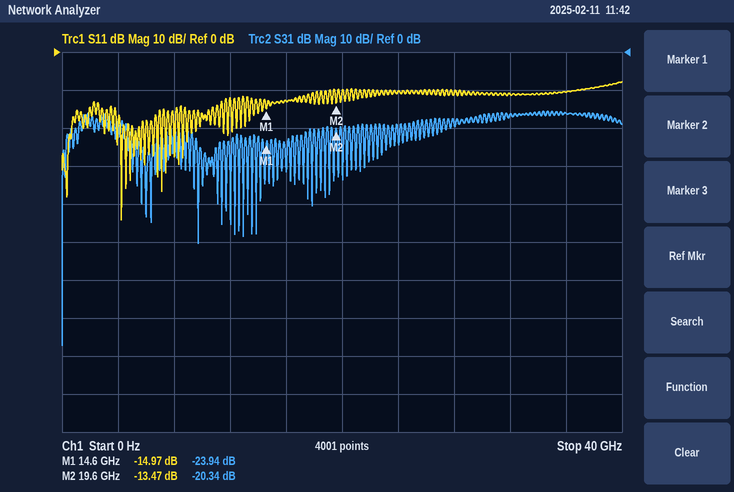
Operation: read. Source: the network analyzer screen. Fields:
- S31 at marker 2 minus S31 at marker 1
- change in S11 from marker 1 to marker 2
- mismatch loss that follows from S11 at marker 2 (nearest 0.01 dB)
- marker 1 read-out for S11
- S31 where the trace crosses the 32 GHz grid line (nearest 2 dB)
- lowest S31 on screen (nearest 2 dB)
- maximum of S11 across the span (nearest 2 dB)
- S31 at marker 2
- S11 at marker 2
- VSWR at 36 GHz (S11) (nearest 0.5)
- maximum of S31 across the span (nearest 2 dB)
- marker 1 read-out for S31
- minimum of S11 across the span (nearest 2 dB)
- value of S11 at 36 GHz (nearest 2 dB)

3.60 dB
1.50 dB
0.20 dB
-14.97 dB
-16 dB
-78 dB
-8 dB
-20.34 dB
-13.47 dB
2.0
-16 dB
-23.94 dB
-44 dB
-10 dB
